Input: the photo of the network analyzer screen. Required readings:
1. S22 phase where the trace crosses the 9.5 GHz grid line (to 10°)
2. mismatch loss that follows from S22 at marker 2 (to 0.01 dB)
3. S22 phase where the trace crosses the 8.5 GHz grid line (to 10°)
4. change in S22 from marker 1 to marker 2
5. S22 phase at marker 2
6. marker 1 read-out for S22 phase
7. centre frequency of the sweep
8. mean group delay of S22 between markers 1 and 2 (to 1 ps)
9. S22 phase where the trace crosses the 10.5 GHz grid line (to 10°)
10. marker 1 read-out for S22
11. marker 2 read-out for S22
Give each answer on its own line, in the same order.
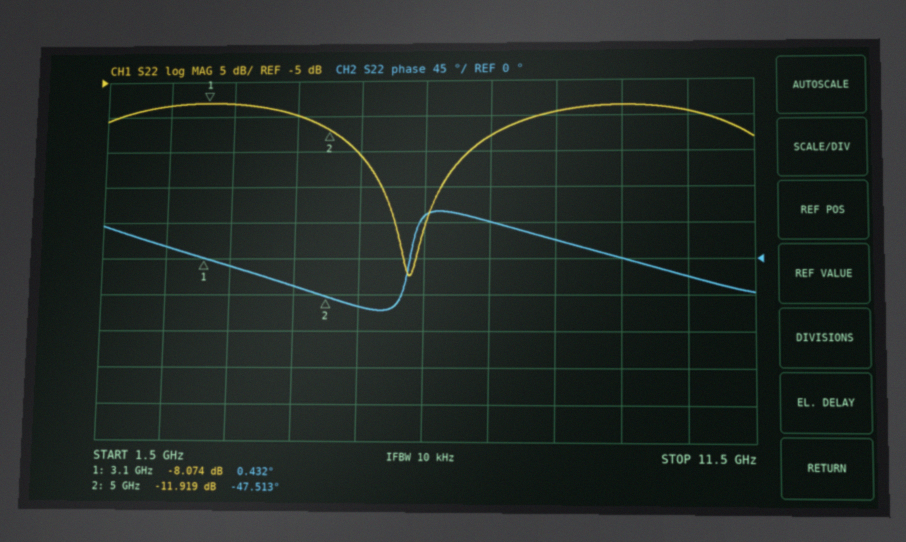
0°
0.29 dB
20°
-3.845 dB
-47.513°
0.432°
6.5 GHz
70 ps
-20°
-8.074 dB
-11.919 dB
